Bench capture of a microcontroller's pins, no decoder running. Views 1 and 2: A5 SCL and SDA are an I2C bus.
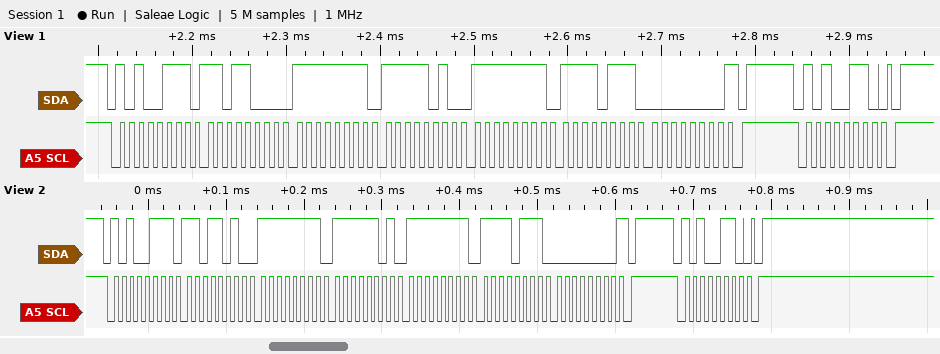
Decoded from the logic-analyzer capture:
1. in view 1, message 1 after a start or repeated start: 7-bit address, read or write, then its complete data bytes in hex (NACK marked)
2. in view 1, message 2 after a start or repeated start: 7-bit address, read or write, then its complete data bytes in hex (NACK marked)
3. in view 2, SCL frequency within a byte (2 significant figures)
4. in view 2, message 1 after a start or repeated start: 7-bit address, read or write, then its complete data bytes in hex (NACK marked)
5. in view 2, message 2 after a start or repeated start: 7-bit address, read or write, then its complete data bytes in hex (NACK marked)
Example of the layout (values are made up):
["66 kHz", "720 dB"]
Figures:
["0x53 read: D8 FF FA FF F7 00 NACK", "0x53 write", "100 kHz", "0x53 read: DA FF FD FF F7 00 NACK", "0x53 write"]
